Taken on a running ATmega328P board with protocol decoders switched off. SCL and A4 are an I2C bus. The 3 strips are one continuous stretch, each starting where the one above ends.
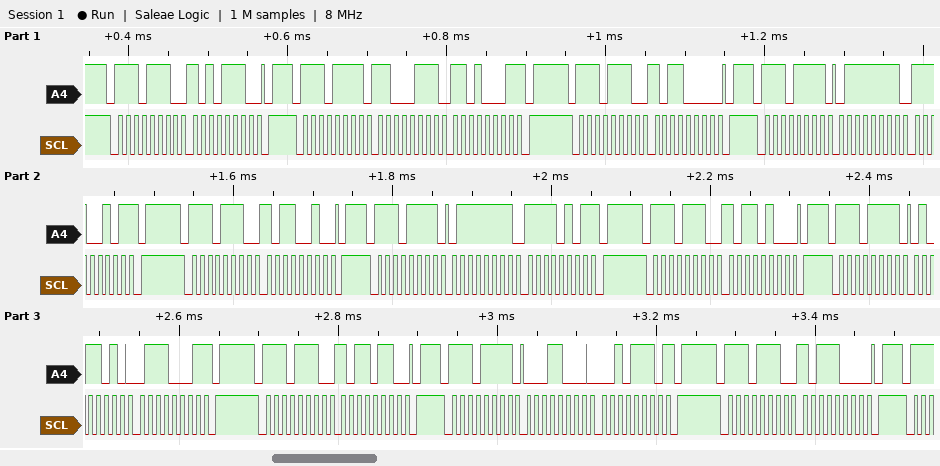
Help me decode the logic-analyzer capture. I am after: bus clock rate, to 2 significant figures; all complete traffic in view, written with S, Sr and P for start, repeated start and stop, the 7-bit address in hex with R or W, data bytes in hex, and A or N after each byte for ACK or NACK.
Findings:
100 kHz
S 77W A AE A P S 77R A C7 A D1 N P S 77W A B0 A P S 77R A 7F A E5 N P S 77W A B2 A P S 77R A 7F A F5 N P S 77W A B4 A P S 77R A 5A A 71 N P S 77W A B6 A P S 77R A 18 A 2E N P S 77W A B8 A P
